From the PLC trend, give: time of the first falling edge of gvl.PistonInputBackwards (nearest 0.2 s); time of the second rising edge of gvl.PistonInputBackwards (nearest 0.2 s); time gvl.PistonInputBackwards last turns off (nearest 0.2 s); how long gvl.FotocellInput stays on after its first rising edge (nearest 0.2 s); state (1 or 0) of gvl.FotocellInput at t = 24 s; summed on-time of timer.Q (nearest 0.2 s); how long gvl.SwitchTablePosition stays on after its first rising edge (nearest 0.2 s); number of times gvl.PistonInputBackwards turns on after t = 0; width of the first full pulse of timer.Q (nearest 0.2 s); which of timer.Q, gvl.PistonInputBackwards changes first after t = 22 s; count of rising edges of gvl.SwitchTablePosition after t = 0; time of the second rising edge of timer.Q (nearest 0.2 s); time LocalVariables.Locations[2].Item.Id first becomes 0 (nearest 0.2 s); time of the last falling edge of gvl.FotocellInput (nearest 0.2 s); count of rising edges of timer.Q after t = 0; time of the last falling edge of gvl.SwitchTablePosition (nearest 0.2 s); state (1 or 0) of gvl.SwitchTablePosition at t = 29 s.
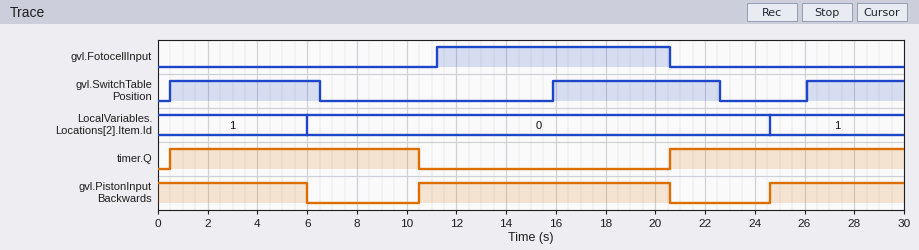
6.0 s
24.6 s
20.6 s
9.4 s
0
19.4 s
6.0 s
2
10.0 s
gvl.PistonInputBackwards
3
20.6 s
6.0 s
20.6 s
2
22.6 s
1
